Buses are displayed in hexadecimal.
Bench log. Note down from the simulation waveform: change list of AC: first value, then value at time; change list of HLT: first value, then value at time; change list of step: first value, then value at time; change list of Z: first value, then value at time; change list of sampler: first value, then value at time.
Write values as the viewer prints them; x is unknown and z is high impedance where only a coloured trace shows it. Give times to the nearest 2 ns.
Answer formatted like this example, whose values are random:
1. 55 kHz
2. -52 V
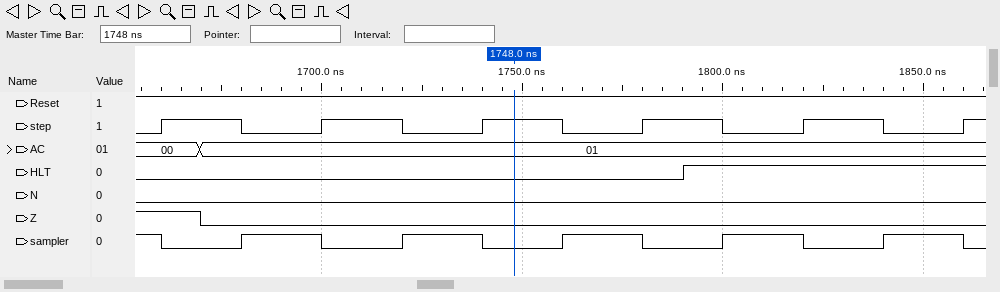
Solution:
1. 00, 01 at 1670 ns
2. 0, 1 at 1790 ns
3. 0, 1 at 1660 ns, 0 at 1680 ns, 1 at 1700 ns, 0 at 1720 ns, 1 at 1740 ns, 0 at 1760 ns, 1 at 1780 ns, 0 at 1800 ns, 1 at 1820 ns, 0 at 1840 ns, 1 at 1860 ns
4. 1, 0 at 1670 ns
5. 1, 0 at 1660 ns, 1 at 1680 ns, 0 at 1700 ns, 1 at 1720 ns, 0 at 1740 ns, 1 at 1760 ns, 0 at 1780 ns, 1 at 1800 ns, 0 at 1820 ns, 1 at 1840 ns, 0 at 1860 ns
